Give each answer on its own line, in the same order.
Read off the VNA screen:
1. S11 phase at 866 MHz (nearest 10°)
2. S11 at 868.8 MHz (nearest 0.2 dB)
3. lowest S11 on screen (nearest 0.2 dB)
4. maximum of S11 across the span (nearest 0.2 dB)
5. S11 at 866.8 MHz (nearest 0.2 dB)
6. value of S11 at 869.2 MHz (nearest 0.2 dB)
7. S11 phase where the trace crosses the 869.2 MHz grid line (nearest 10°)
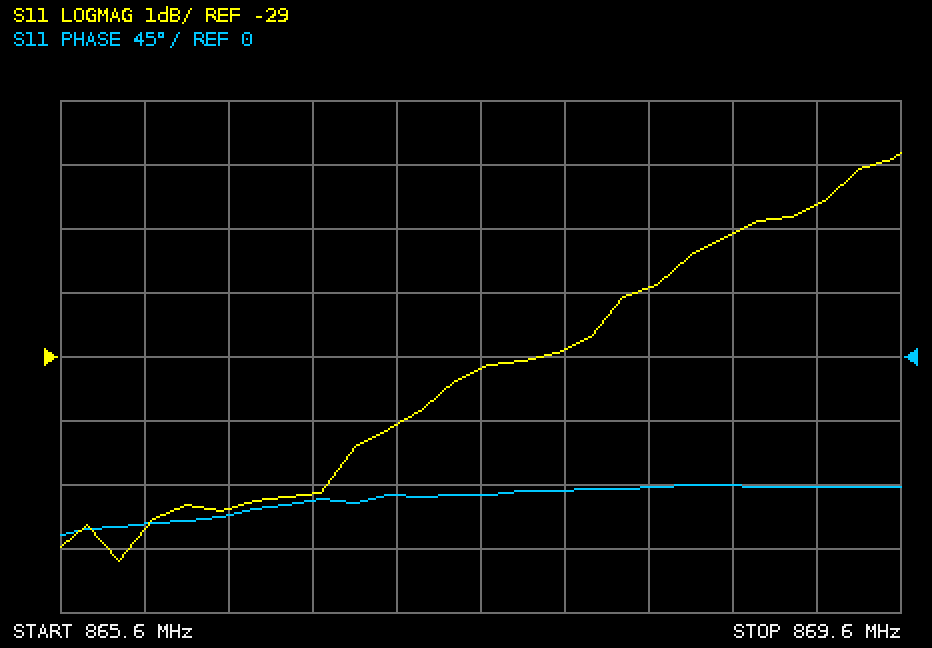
-120°
-27.0 dB
-32.2 dB
-25.8 dB
-31.2 dB
-26.6 dB
-90°
